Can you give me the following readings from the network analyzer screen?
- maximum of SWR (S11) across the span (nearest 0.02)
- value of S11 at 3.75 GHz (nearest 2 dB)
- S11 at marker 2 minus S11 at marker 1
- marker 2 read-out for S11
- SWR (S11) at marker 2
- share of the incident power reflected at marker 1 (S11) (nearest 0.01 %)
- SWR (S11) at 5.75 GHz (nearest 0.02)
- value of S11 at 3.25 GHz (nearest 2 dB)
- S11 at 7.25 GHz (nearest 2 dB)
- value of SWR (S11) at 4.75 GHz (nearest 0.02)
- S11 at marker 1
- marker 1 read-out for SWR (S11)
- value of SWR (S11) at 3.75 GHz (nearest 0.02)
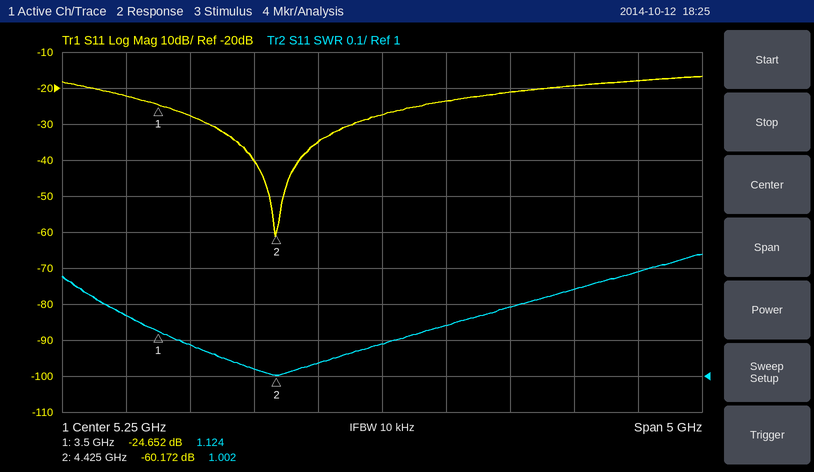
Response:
1.34
-28 dB
-35.520 dB
-60.172 dB
1.002
0.34 %
1.14
-22 dB
-18 dB
1.04
-24.652 dB
1.124
1.08
